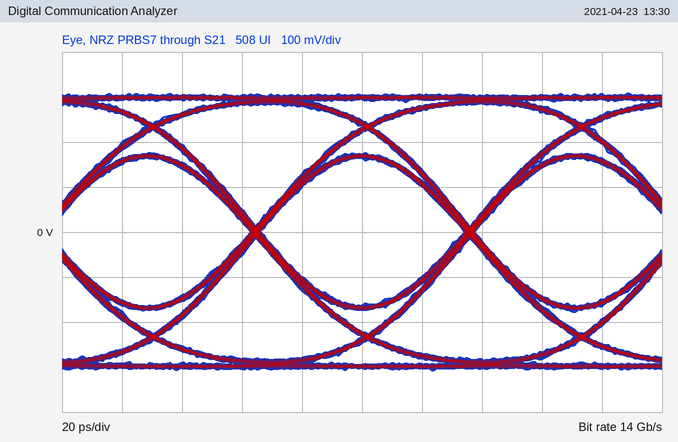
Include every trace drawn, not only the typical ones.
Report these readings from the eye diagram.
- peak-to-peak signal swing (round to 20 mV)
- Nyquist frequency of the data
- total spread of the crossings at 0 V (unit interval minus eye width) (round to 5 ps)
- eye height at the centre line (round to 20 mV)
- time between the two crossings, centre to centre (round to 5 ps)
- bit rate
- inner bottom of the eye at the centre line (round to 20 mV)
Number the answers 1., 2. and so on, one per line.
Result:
1. 620 mV
2. 7 GHz
3. 5 ps
4. 320 mV
5. 70 ps
6. 14 Gb/s
7. -160 mV
